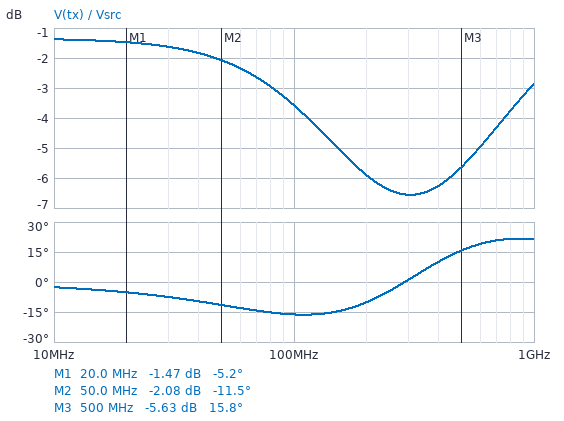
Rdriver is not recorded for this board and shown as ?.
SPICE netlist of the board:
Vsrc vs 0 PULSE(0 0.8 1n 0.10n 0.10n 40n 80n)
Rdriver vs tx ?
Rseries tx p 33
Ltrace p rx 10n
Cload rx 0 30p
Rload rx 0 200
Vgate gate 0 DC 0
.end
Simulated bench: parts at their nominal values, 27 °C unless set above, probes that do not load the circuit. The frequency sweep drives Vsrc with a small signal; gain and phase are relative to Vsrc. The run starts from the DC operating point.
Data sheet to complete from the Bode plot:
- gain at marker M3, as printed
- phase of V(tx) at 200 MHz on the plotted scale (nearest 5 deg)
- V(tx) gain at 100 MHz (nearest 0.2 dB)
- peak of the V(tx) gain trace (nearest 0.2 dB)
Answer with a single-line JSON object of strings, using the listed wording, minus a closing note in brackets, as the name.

{"gain at marker M3, as printed": "-5.63 dB", "phase of V(tx) at 200 MHz on the plotted scale": "-10 deg", "V(tx) gain at 100 MHz": "-3.6 dB", "peak of the V(tx) gain trace": "-1.4 dB"}
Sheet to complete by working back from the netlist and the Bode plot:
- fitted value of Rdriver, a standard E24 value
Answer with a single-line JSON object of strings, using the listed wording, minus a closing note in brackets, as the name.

{"fitted value of Rdriver, a standard E24 value": "39 Ω"}
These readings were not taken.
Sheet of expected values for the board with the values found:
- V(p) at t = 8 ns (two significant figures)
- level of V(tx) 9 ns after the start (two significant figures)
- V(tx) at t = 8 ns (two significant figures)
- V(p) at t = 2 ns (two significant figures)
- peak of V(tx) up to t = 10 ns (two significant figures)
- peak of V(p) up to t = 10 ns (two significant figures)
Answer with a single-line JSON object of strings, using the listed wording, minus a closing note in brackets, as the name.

{"V(p) at t = 8 ns": "580 mV", "level of V(tx) 9 ns after the start": "680 mV", "V(tx) at t = 8 ns": "680 mV", "V(p) at t = 2 ns": "210 mV", "peak of V(tx) up to t = 10 ns": "680 mV", "peak of V(p) up to t = 10 ns": "590 mV"}
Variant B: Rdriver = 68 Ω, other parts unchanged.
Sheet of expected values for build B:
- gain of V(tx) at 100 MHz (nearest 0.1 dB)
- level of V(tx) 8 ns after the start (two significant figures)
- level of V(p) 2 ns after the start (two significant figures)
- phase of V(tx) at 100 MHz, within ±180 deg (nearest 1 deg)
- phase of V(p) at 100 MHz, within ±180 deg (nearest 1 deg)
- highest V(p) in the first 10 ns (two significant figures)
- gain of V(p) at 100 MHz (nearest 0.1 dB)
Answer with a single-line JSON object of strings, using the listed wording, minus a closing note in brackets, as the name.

{"gain of V(tx) at 100 MHz": "-5.7 dB", "level of V(tx) 8 ns after the start": "610 mV", "level of V(p) 2 ns after the start": "170 mV", "phase of V(tx) at 100 MHz, within ±180 deg": "-22 deg", "phase of V(p) at 100 MHz, within ±180 deg": "-52 deg", "highest V(p) in the first 10 ns": "530 mV", "gain of V(p) at 100 MHz": "-8.6 dB"}
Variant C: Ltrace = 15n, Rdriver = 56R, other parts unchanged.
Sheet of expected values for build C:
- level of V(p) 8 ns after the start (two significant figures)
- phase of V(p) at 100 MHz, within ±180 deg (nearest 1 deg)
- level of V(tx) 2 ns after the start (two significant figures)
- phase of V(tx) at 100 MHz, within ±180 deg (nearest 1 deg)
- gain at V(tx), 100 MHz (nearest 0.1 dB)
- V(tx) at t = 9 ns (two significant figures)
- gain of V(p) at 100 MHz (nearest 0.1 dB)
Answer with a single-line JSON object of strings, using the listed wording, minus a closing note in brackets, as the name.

{"level of V(p) 8 ns after the start": "540 mV", "phase of V(p) at 100 MHz, within ±180 deg": "-50 deg", "level of V(tx) 2 ns after the start": "400 mV", "phase of V(tx) at 100 MHz, within ±180 deg": "-20 deg", "gain at V(tx), 100 MHz": "-5.1 dB", "V(tx) at t = 9 ns": "640 mV", "gain of V(p) at 100 MHz": "-8.3 dB"}
